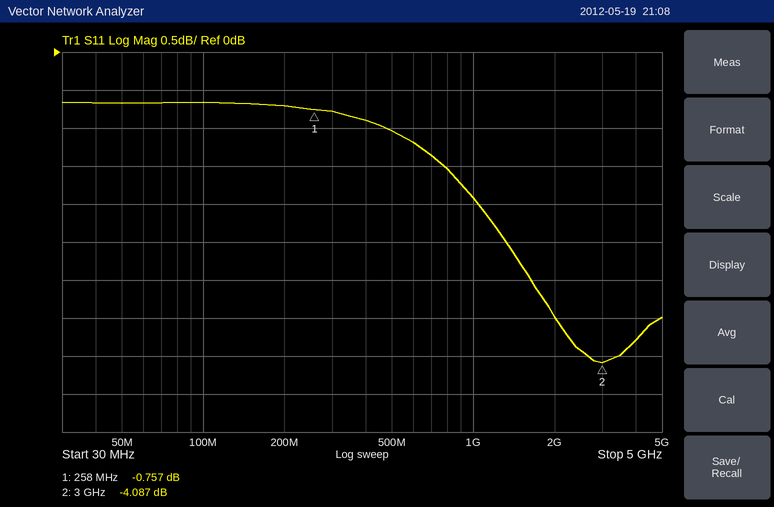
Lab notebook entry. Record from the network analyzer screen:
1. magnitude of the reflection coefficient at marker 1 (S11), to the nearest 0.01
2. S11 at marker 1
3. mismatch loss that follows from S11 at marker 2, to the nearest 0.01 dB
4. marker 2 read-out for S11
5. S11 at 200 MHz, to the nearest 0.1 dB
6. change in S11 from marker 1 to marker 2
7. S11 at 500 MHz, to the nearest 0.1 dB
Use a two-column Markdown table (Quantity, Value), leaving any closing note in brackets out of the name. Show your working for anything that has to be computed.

| Quantity | Value |
|---|---|
| magnitude of the reflection coefficient at marker 1 (S11), to the nearest 0.01 | 10^(-0.757/20) ≈ 0.92 |
| S11 at marker 1 | -0.757 dB |
| mismatch loss that follows from S11 at marker 2, to the nearest 0.01 dB | −10 log10(1 − 10^(-4.087/10)) ≈ 2.15 dB |
| marker 2 read-out for S11 | -4.087 dB |
| S11 at 200 MHz, to the nearest 0.1 dB | -0.7 dB |
| change in S11 from marker 1 to marker 2 | -4.087 − (-0.757) = -3.330 dB |
| S11 at 500 MHz, to the nearest 0.1 dB | -1.0 dB |
